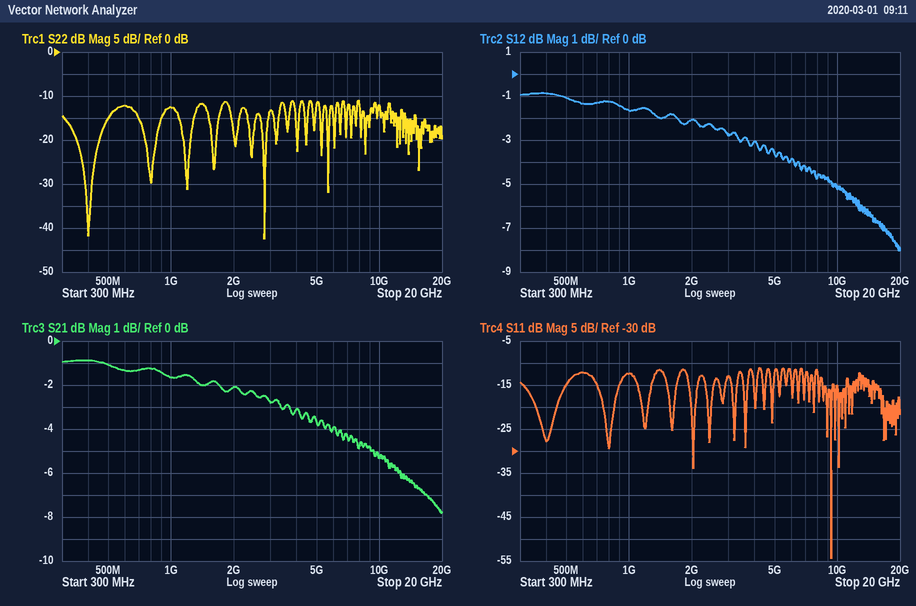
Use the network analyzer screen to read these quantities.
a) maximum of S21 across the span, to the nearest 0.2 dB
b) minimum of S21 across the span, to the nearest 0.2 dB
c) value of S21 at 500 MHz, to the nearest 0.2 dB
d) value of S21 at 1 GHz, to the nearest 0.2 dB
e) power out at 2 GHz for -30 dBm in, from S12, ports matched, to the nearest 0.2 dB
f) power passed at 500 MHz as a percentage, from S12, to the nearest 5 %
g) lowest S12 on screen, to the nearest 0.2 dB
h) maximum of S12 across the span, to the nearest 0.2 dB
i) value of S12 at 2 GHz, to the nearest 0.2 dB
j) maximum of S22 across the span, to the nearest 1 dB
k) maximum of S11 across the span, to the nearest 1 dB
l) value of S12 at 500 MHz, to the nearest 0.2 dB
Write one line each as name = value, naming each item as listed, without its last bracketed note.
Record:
maximum of S21 across the span, to the nearest 0.2 dB = -0.8 dB
minimum of S21 across the span, to the nearest 0.2 dB = -7.8 dB
value of S21 at 500 MHz, to the nearest 0.2 dB = -1.0 dB
value of S21 at 1 GHz, to the nearest 0.2 dB = -1.6 dB
power out at 2 GHz for -30 dBm in, from S12, ports matched, to the nearest 0.2 dB = -32.0 dBm
power passed at 500 MHz as a percentage, from S12, to the nearest 5 % = 80 %
lowest S12 on screen, to the nearest 0.2 dB = -8.0 dB
maximum of S12 across the span, to the nearest 0.2 dB = -0.8 dB
value of S12 at 2 GHz, to the nearest 0.2 dB = -2.0 dB
maximum of S22 across the span, to the nearest 1 dB = -11 dB
maximum of S11 across the span, to the nearest 1 dB = -11 dB
value of S12 at 500 MHz, to the nearest 0.2 dB = -1.0 dB
